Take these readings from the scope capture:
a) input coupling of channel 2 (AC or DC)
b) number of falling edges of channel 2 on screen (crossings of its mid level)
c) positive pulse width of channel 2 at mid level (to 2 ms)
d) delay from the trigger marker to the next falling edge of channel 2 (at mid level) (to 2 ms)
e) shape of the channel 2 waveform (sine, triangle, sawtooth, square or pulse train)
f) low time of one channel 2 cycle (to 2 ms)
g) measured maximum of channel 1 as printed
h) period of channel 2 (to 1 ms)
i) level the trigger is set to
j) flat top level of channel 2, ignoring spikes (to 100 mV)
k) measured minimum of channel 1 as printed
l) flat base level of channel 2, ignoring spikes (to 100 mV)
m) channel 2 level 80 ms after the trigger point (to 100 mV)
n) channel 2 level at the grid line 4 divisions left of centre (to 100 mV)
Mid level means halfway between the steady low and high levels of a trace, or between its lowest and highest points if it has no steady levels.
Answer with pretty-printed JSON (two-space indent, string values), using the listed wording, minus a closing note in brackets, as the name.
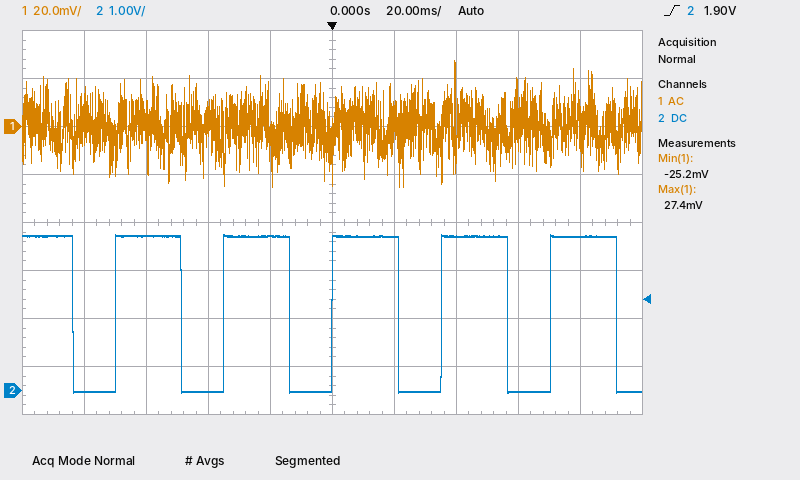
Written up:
{
  "input coupling of channel 2": "DC",
  "number of falling edges of channel 2 on screen": "6",
  "positive pulse width of channel 2 at mid level": "22 ms",
  "delay from the trigger marker to the next falling edge of channel 2 (at mid level)": "22 ms",
  "shape of the channel 2 waveform": "pulse train",
  "low time of one channel 2 cycle": "14 ms",
  "measured maximum of channel 1 as printed": "27.4 mV",
  "period of channel 2": "35 ms",
  "level the trigger is set to": "1.90 V",
  "flat top level of channel 2, ignoring spikes": "3.2 V",
  "measured minimum of channel 1 as printed": "-25.2 mV",
  "flat base level of channel 2, ignoring spikes": "0.0 V",
  "channel 2 level 80 ms after the trigger point": "3.2 V",
  "channel 2 level at the grid line 4 divisions left of centre": "0.0 V"
}
